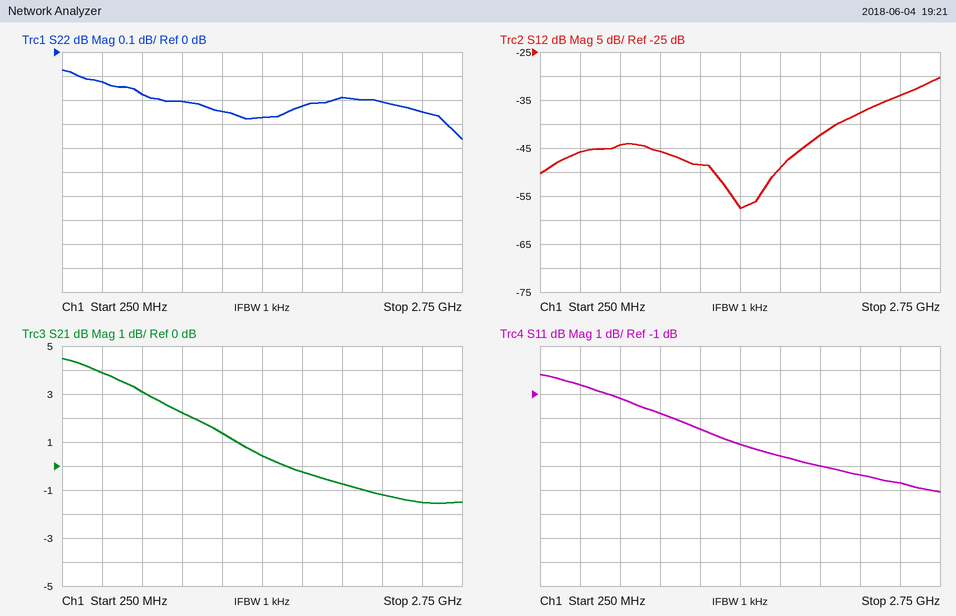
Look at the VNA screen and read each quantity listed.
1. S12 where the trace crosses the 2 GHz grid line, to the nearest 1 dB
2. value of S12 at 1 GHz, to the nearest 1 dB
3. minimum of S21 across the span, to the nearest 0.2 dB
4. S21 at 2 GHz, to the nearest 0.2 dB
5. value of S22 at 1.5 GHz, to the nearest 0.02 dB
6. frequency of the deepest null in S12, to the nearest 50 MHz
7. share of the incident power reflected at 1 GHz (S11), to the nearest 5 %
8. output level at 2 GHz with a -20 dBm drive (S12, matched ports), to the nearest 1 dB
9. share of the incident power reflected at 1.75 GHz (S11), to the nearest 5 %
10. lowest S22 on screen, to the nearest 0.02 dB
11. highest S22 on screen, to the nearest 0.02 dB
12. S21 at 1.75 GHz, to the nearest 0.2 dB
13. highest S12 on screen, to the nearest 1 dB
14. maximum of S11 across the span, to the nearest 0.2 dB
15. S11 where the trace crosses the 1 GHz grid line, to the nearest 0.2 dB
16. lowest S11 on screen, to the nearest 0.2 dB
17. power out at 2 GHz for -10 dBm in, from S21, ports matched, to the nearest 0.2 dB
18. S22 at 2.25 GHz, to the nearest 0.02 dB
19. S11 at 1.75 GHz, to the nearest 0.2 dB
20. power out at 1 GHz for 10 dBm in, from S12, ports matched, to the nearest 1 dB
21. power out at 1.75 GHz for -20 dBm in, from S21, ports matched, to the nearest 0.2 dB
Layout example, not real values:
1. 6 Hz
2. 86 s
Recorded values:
1. -42 dB
2. -46 dB
3. -1.6 dB
4. -0.8 dB
5. -0.28 dB
6. 1.50 GHz
7. 65 %
8. -62 dBm
9. 45 %
10. -0.36 dB
11. -0.08 dB
12. -0.2 dB
13. -30 dB
14. -0.2 dB
15. -1.8 dB
16. -5.0 dB
17. -10.8 dBm
18. -0.20 dB
19. -3.6 dB
20. -36 dBm
21. -20.2 dBm
